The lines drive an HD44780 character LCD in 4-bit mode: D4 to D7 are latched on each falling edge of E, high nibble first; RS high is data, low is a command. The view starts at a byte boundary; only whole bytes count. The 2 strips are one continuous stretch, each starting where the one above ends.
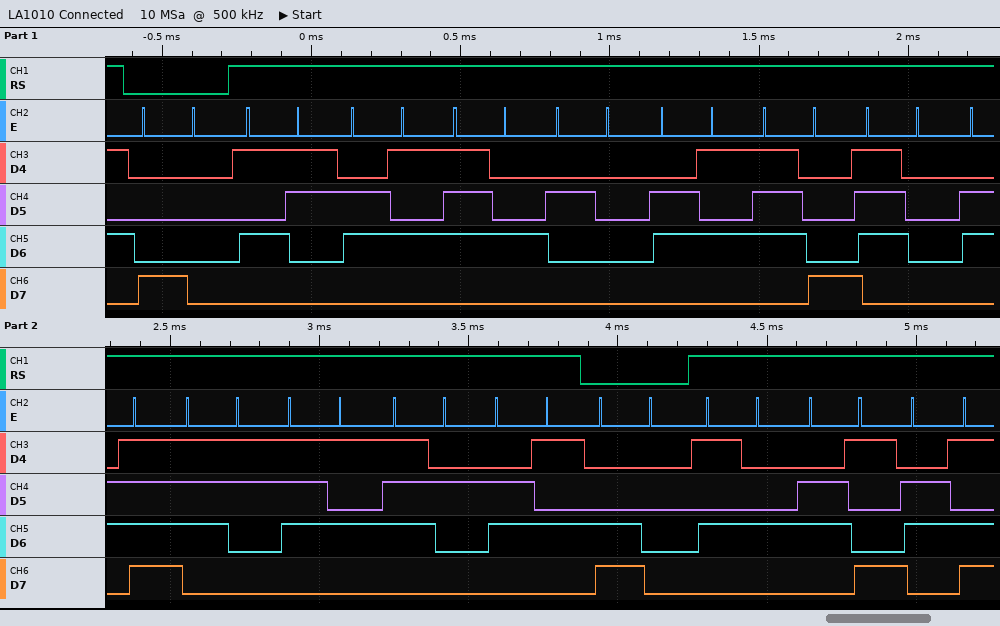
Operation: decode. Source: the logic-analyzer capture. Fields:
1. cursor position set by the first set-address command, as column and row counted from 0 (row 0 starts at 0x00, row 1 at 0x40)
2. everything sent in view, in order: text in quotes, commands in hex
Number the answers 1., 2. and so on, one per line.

1. column 0, row 0
2. 0x80 "Set exposure" 0xC0 "Tim"
